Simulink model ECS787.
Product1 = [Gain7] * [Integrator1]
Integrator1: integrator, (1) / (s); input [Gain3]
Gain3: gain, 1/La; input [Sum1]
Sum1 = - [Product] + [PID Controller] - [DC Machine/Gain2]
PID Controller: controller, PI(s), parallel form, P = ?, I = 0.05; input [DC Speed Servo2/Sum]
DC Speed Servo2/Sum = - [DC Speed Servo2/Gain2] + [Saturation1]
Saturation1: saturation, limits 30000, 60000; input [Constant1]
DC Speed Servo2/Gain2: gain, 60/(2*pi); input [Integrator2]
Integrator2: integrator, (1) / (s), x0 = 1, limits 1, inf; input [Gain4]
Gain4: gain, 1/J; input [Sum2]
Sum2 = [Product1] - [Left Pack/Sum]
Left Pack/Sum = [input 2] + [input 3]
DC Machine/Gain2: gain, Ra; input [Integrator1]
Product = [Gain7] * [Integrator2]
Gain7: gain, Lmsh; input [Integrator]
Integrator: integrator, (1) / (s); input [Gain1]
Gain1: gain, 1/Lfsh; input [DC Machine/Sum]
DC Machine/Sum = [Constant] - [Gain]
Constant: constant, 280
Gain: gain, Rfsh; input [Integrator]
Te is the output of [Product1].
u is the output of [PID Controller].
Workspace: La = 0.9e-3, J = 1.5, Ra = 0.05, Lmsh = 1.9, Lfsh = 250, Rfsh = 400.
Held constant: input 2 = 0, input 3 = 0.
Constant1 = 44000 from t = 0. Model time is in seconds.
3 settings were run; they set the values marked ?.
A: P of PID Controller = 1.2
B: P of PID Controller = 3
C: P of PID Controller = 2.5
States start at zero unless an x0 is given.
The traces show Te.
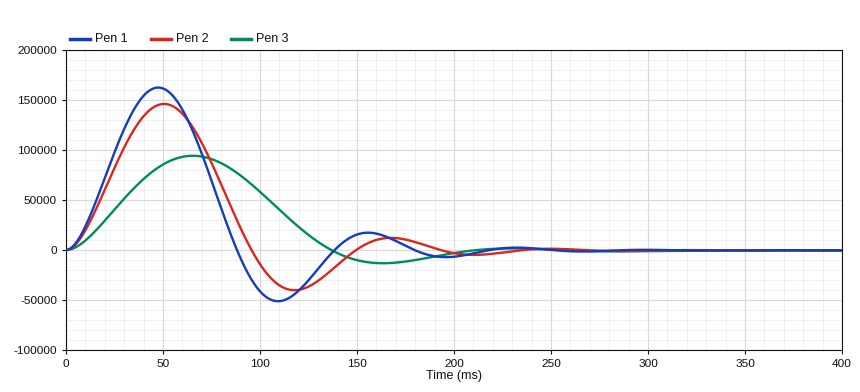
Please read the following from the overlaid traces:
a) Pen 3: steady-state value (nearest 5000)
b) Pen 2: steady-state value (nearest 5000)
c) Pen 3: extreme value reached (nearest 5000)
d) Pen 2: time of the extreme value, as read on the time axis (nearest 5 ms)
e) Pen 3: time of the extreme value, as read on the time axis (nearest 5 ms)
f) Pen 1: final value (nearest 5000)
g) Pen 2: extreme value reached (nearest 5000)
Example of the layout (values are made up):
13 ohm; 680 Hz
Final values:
0; 0; 95000; 50 ms; 65 ms; 0; 145000
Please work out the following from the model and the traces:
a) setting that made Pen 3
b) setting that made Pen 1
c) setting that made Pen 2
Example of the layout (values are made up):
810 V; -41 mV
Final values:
A; B; C
